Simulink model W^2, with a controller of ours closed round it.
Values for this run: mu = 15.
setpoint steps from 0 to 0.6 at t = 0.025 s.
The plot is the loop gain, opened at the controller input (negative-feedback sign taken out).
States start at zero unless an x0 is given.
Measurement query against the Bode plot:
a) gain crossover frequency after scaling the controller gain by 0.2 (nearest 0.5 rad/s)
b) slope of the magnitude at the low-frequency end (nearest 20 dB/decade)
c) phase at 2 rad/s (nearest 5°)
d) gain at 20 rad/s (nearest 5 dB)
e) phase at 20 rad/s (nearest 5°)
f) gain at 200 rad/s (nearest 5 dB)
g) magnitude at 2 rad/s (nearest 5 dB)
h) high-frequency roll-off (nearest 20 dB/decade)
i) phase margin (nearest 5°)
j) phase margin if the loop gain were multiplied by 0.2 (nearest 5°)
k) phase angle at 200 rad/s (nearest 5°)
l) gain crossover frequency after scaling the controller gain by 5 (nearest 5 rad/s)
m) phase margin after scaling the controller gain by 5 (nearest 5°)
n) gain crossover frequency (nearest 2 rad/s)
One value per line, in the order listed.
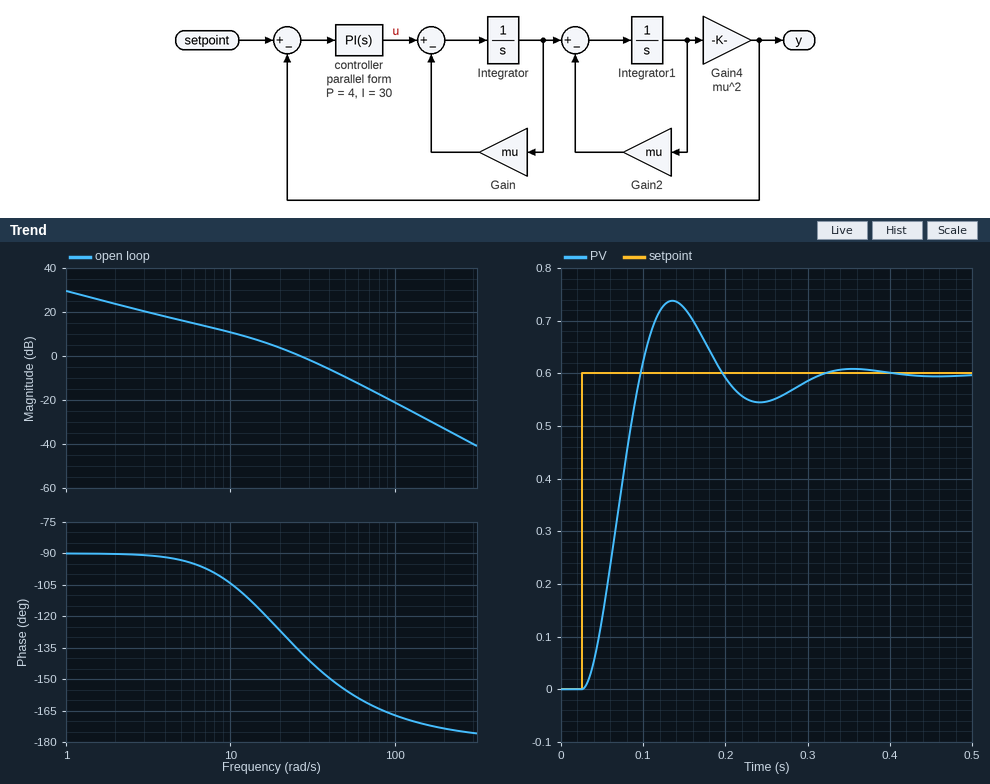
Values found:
6.5 rad/s
-20 dB/decade
-90°
5 dB
-125°
-35 dB
25 dB
-40 dB/decade
45°
85°
-175°
65 rad/s
20°
26 rad/s
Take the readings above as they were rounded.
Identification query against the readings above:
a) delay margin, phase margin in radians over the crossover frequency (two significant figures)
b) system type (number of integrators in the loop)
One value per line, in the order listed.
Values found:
0.030 s
1
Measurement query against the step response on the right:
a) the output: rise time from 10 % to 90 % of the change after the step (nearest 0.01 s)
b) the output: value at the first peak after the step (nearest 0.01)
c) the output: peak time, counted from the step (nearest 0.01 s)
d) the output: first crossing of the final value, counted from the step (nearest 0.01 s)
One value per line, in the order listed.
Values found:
0.05 s
0.74
0.11 s
0.07 s
